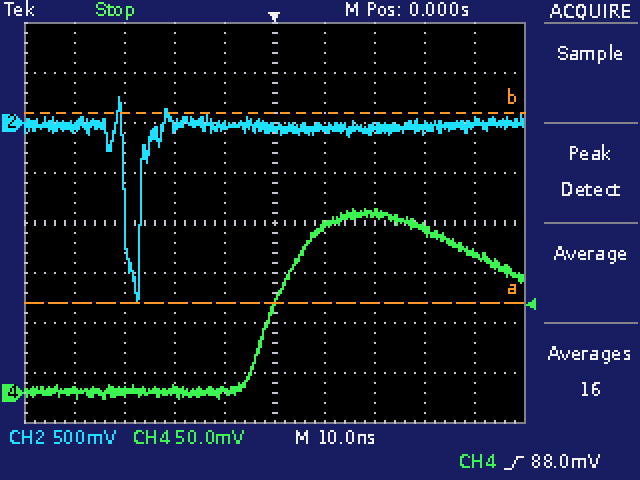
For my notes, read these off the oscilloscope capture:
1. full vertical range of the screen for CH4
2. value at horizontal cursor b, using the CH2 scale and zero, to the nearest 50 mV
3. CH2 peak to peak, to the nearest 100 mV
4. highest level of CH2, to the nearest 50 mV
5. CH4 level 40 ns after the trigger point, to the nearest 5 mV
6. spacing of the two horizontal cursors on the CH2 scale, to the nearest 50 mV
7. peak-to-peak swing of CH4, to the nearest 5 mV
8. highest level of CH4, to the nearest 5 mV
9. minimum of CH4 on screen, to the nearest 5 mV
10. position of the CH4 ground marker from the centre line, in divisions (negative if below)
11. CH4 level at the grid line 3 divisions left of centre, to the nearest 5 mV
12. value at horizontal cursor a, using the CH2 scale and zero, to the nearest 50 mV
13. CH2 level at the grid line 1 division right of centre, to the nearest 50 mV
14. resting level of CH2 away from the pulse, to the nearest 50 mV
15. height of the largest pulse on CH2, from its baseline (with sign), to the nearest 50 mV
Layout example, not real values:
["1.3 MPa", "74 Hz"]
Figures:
["400 mV", "100 mV", "2.00 V", "250 mV", "140 mV", "1.90 V", "190 mV", "185 mV", "-5 mV", "-3.4 div", "0 mV", "-1.80 V", "-50 mV", "-50 mV", "-1.75 V"]
